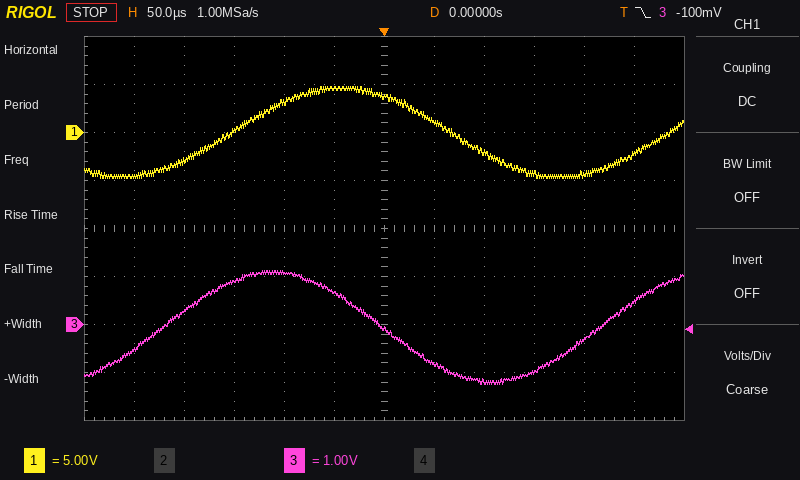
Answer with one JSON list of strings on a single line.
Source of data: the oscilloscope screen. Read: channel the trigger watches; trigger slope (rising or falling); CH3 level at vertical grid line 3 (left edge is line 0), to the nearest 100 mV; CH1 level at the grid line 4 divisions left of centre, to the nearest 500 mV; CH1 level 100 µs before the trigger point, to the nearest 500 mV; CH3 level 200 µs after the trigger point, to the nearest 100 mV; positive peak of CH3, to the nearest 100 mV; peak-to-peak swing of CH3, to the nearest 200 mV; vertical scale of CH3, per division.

["CH3", "falling", "900 mV", "-3.0 V", "3.0 V", "-300 mV", "1.1 V", "2.4 V", "1 V"]
